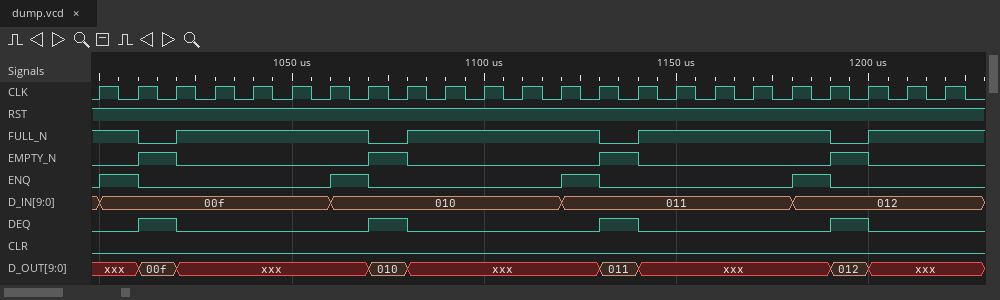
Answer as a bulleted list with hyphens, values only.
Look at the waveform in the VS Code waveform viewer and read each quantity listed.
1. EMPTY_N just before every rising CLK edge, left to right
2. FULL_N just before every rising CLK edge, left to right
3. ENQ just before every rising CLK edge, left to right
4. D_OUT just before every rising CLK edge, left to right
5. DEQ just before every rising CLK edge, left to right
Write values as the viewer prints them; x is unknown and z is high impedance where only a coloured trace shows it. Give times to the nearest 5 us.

- 0 0 1 0 0 0 0 0 1 0 0 0 0 0 1 0 0 0 0 0 1 0 0
- 1 1 0 1 1 1 1 1 0 1 1 1 1 1 0 1 1 1 1 1 0 1 1
- 0 1 0 0 0 0 0 1 0 0 0 0 0 1 0 0 0 0 0 1 0 0 0
- xxx, xxx, 00f, xxx, xxx, xxx, xxx, xxx, 010, xxx, xxx, xxx, xxx, xxx, 011, xxx, xxx, xxx, xxx, xxx, 012, xxx, xxx
- 0 0 1 0 0 0 0 0 1 0 0 0 0 0 1 0 0 0 0 0 1 0 0
